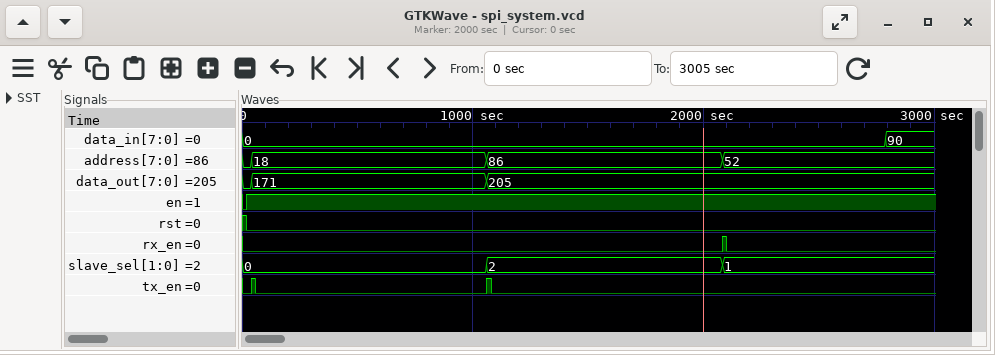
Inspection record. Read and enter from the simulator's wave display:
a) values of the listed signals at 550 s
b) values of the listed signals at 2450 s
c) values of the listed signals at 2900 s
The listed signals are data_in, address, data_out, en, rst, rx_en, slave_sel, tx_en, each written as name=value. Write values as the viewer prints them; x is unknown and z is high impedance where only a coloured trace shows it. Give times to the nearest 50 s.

data_in=0, address=18, data_out=171, en=1, rst=0, rx_en=0, slave_sel=0, tx_en=0
data_in=0, address=52, data_out=205, en=1, rst=0, rx_en=0, slave_sel=1, tx_en=0
data_in=90, address=52, data_out=205, en=1, rst=0, rx_en=0, slave_sel=1, tx_en=0
